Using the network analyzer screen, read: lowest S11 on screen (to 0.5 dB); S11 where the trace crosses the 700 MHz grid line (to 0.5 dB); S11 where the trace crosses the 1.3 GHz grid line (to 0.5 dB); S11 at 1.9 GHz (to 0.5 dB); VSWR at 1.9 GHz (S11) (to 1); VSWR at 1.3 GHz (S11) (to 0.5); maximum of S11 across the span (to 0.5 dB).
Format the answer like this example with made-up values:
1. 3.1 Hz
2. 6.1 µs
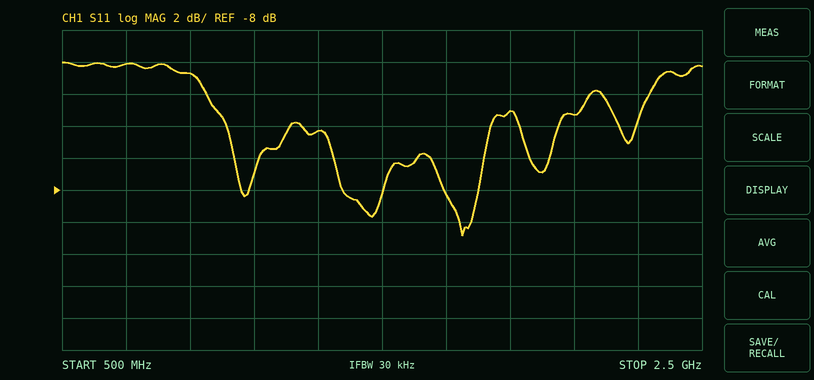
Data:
1. -11.0 dB
2. 0.0 dB
3. -4.5 dB
4. -3.0 dB
5. 6
6. 4.0
7. 0.0 dB
